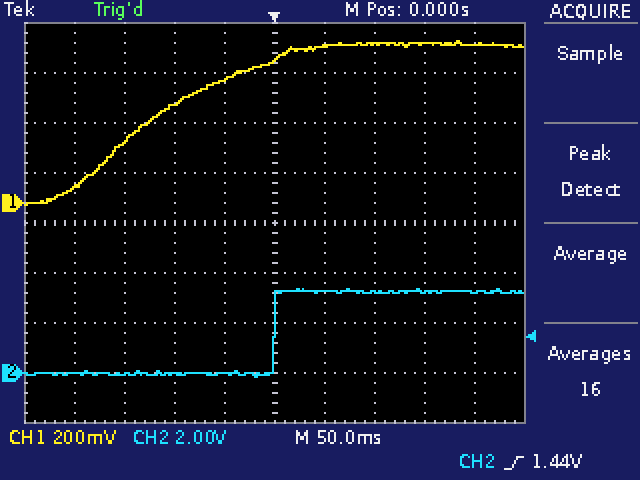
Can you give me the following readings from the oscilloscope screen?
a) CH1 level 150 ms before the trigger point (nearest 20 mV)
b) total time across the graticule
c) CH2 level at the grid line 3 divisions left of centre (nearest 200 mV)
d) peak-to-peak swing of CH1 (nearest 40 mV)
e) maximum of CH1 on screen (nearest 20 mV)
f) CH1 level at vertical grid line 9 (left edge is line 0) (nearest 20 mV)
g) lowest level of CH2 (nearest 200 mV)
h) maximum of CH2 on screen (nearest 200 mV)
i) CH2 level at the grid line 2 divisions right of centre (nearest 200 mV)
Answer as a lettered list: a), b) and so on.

a) 240 mV
b) 500 ms
c) 0.0 V
d) 640 mV
e) 640 mV
f) 640 mV
g) -200 mV
h) 3.4 V
i) 3.2 V
